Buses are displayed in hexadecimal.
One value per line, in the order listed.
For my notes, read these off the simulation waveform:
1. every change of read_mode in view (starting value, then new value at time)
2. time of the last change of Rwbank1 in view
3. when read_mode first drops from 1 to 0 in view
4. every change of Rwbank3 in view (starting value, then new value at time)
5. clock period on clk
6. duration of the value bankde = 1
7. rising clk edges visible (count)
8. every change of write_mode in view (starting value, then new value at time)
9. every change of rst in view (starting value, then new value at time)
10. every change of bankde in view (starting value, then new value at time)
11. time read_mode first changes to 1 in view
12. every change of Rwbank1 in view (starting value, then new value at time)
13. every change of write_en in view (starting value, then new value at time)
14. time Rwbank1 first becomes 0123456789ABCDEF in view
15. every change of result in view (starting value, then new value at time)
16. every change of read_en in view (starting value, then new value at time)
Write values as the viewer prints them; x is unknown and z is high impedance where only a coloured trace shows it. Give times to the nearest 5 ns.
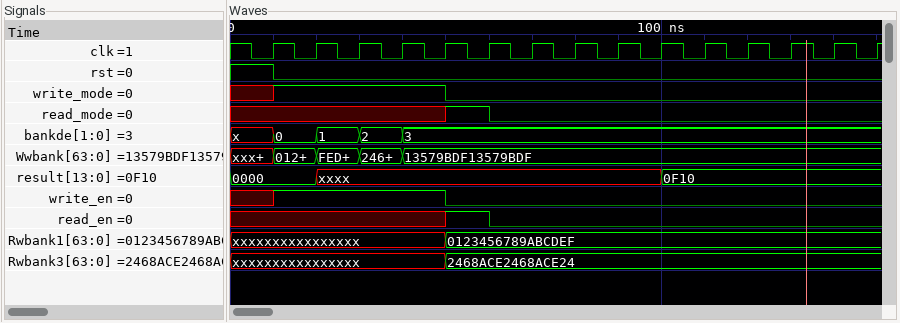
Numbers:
x, 1 at 50 ns, 0 at 60 ns
50 ns
60 ns
xxxxxxxxxxxxxxxx, 2468ACE2468ACE24 at 50 ns
10 ns
10 ns
15
x, 1 at 10 ns, 0 at 50 ns
1, 0 at 10 ns
x, 0 at 10 ns, 1 at 20 ns, 2 at 30 ns, 3 at 40 ns
50 ns
xxxxxxxxxxxxxxxx, 0123456789ABCDEF at 50 ns
x, 1 at 10 ns, 0 at 50 ns
50 ns
0000, xxxx at 20 ns, 0F10 at 100 ns
x, 1 at 50 ns, 0 at 60 ns
